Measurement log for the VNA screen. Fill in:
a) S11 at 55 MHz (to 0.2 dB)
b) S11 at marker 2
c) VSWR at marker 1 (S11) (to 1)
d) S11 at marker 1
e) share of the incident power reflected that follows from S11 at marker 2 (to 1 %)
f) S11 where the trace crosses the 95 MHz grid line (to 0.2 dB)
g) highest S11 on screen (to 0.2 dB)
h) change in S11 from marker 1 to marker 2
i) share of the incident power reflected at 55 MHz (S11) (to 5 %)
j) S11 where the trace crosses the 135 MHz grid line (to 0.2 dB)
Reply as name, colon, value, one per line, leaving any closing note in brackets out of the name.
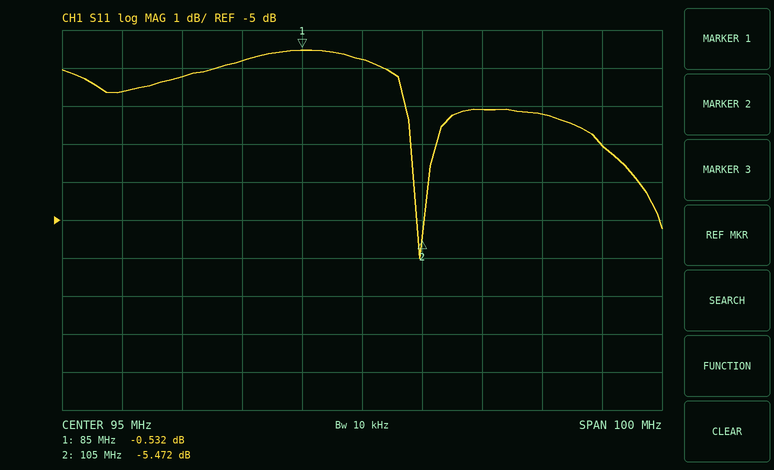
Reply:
S11 at 55 MHz: -1.6 dB
S11 at marker 2: -5.472 dB
VSWR at marker 1 (S11): 33
S11 at marker 1: -0.532 dB
share of the incident power reflected that follows from S11 at marker 2: 28 %
S11 where the trace crosses the 95 MHz grid line: -0.8 dB
highest S11 on screen: -0.6 dB
change in S11 from marker 1 to marker 2: -4.940 dB
share of the incident power reflected at 55 MHz (S11): 70 %
S11 where the trace crosses the 135 MHz grid line: -3.0 dB
